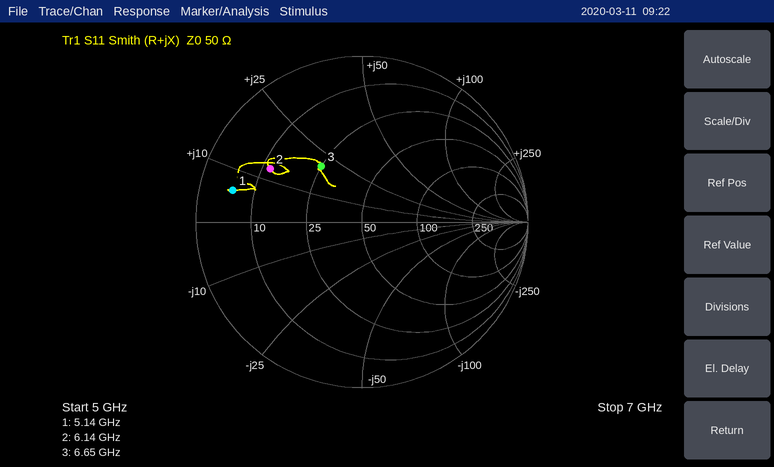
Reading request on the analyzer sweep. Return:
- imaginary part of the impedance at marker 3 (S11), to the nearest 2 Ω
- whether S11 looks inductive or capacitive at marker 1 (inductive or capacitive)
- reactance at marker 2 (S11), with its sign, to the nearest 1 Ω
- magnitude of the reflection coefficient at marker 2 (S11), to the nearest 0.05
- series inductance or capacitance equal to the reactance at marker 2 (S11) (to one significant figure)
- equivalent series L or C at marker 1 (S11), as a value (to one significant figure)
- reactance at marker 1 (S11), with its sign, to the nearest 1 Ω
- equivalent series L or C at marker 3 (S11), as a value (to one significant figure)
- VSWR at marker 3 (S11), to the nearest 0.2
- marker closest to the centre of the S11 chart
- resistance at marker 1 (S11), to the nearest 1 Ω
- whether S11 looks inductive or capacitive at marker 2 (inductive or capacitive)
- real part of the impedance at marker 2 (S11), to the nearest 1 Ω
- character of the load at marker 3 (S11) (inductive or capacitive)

+20 Ω
inductive
+13 Ω
0.65
300 pH
200 pH
+6 Ω
500 pH
2.4
marker 3
6 Ω
inductive
12 Ω
inductive
